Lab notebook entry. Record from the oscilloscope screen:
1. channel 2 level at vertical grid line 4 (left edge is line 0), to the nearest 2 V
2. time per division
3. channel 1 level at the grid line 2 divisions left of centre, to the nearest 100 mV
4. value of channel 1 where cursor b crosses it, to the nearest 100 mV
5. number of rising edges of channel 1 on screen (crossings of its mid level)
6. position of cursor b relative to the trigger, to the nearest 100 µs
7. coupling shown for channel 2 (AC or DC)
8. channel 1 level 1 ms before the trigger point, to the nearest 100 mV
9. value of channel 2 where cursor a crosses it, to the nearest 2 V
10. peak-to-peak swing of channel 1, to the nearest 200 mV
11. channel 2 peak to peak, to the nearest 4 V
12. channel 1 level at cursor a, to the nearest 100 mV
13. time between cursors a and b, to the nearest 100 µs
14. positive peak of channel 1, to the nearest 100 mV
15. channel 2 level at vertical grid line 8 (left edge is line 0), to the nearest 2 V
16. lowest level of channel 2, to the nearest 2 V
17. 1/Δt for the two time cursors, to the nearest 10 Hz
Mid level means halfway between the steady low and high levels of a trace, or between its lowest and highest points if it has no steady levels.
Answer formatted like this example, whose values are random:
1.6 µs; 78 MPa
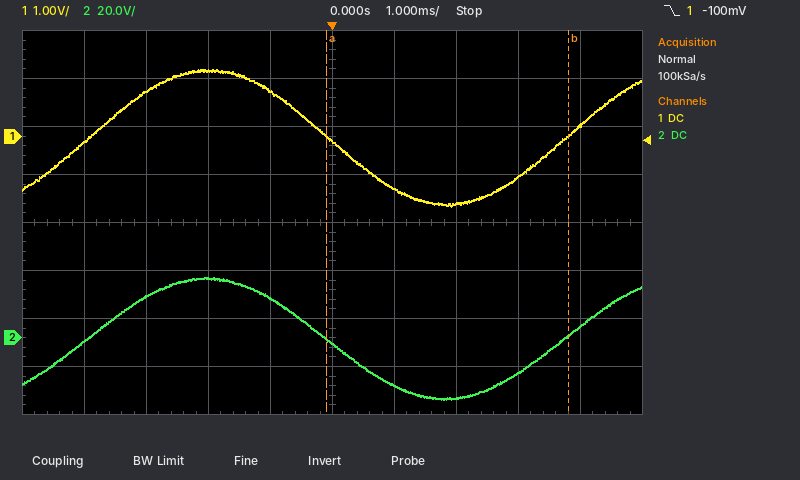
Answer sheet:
16 V; 1 ms; 1.4 V; 0.0 V; 2; +3.8 ms; DC; 900 mV; 0 V; 2.8 V; 52 V; 0.0 V; 3.9 ms; 1.4 V; -14 V; -26 V; 260 Hz
